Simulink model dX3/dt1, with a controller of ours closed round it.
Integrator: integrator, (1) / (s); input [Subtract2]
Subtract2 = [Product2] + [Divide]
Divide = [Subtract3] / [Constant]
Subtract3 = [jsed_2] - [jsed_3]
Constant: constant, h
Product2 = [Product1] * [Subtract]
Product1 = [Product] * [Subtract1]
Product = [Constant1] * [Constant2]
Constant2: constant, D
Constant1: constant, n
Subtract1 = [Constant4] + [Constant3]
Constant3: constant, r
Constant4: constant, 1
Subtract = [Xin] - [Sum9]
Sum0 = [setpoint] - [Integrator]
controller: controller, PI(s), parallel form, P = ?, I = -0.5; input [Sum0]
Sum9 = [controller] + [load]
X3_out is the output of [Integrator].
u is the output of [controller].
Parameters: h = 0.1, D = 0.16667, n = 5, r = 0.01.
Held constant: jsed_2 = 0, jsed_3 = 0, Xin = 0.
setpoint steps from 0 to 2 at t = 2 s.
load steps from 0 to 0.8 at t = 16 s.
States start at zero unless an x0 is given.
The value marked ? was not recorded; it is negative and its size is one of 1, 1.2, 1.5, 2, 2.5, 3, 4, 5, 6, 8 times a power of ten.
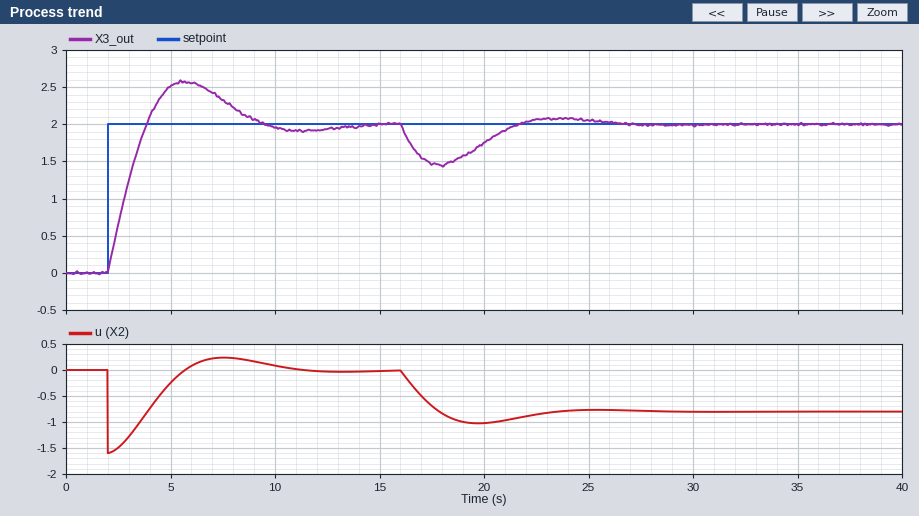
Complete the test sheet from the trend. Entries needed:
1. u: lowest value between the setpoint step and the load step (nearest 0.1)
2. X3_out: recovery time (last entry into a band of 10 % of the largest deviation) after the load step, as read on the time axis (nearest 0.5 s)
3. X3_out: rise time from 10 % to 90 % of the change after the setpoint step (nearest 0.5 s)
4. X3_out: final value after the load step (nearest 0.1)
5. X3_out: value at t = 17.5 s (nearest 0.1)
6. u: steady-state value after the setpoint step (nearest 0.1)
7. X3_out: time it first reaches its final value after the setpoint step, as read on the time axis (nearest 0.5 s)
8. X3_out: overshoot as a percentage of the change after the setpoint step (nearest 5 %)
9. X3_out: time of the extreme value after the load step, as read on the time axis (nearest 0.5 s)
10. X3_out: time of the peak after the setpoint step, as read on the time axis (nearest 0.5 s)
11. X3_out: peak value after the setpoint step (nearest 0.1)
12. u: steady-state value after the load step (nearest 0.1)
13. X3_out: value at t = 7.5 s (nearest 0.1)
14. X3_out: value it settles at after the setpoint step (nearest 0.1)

-1.6
25.0 s
1.5 s
2.0
1.5
0.0
4.0 s
30 %
18.0 s
5.5 s
2.6
-0.8
2.3
2.0
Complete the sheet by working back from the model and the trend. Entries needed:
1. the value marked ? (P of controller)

-0.8
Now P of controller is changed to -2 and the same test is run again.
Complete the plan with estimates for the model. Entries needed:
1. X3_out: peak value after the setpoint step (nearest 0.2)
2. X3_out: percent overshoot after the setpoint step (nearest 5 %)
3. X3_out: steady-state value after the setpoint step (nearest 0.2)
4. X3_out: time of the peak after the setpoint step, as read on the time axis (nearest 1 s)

2.2
10 %
2.0
5 s
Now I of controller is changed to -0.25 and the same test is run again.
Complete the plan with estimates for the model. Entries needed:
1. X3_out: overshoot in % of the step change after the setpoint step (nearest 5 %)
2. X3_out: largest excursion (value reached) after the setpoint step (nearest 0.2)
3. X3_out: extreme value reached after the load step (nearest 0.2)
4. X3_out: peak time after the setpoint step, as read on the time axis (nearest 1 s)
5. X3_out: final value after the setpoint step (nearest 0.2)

20 %
2.4
1.4
7 s
2.0
